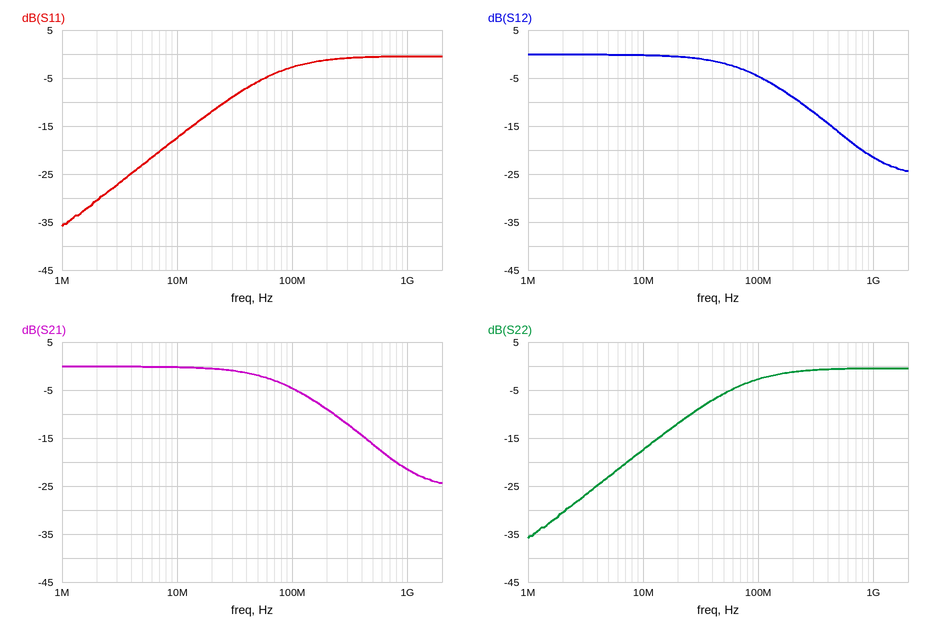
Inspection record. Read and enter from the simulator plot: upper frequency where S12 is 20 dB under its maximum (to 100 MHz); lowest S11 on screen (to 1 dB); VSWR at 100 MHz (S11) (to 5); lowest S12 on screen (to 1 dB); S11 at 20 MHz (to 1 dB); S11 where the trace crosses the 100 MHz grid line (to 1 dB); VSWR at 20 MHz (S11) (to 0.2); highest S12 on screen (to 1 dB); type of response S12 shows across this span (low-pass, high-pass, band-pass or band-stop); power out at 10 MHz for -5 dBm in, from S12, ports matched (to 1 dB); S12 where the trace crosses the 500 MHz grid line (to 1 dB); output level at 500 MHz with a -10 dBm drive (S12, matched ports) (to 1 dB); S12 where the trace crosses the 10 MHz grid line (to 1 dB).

800 MHz
-36 dB
5
-24 dB
-12 dB
-3 dB
1.6
0 dB
low-pass
-5 dBm
-16 dB
-26 dBm
0 dB
